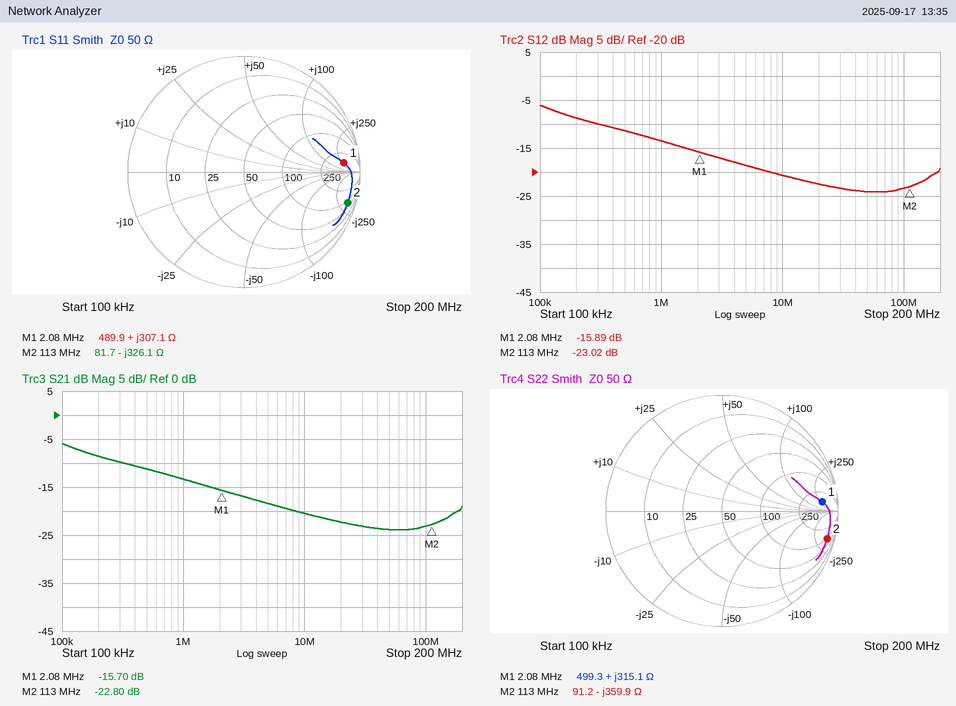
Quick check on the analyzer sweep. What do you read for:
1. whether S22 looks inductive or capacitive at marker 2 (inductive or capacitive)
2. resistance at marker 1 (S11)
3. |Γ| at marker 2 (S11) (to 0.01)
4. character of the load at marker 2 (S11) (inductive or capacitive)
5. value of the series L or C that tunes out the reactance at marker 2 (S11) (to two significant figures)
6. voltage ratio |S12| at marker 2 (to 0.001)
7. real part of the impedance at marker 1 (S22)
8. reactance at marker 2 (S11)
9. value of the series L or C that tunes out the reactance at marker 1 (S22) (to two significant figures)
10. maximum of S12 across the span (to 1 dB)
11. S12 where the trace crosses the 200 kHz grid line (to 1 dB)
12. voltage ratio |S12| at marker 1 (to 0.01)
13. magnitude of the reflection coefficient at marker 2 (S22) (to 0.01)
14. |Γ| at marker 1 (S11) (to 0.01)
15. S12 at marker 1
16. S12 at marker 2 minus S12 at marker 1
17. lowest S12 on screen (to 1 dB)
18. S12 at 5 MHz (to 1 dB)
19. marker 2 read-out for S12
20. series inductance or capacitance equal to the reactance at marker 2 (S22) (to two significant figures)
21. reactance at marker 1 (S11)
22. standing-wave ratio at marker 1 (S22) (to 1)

capacitive
489.9 Ω
0.93
capacitive
460 nH
0.071
499.3 Ω
-326.1 Ω
240 pF
-6 dB
-9 dB
0.16
0.94
0.86
-15.89 dB
-7.13 dB
-24 dB
-19 dB
-23.02 dB
3.9 pF
+307.1 Ω
14
